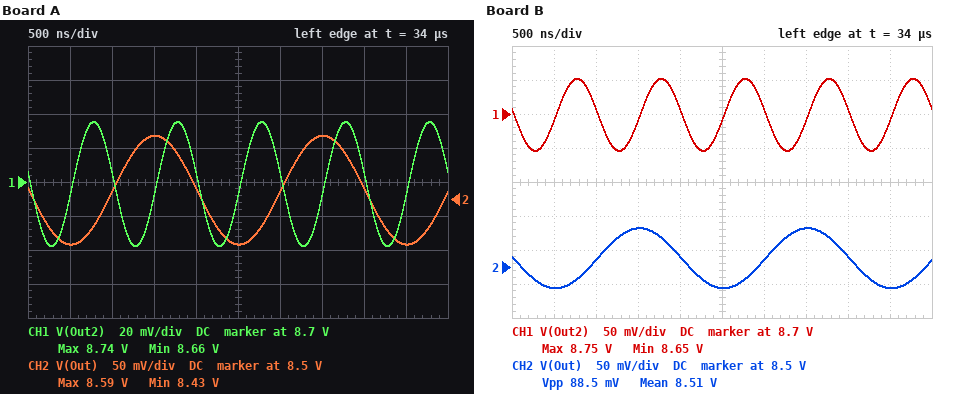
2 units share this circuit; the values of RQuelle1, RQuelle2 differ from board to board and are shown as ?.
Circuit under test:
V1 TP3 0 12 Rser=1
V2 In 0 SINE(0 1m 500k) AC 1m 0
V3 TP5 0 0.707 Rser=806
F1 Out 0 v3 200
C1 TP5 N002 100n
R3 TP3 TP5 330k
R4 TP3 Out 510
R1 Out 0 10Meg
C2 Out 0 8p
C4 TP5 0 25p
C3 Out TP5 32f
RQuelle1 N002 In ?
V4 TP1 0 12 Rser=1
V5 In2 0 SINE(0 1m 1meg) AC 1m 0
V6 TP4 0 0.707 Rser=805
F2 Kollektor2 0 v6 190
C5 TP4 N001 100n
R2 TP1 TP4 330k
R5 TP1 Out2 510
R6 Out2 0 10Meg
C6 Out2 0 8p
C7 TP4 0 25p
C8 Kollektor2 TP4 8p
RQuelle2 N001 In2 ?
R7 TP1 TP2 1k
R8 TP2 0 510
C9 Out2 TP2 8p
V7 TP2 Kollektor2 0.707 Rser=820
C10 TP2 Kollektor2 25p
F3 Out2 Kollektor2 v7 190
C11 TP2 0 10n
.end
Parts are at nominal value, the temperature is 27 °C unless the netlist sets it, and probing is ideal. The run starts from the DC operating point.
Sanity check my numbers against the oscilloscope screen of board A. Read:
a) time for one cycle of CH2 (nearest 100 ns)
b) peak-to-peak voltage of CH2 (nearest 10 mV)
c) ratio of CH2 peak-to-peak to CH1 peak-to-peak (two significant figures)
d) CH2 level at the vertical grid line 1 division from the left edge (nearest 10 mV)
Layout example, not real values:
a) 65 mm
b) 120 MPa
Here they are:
a) 2.0 µs
b) 160 mV
c) 2.2
d) 8.43 V
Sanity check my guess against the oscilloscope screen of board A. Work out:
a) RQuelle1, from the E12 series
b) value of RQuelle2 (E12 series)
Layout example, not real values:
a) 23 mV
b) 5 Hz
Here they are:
a) 470 Ω
b) 1.8 kΩ
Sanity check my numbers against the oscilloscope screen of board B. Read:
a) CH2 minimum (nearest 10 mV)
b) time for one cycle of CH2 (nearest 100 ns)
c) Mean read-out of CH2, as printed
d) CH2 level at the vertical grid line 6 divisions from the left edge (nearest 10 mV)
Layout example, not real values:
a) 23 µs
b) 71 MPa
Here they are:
a) 8.47 V
b) 2.0 µs
c) 8.51 V
d) 8.51 V
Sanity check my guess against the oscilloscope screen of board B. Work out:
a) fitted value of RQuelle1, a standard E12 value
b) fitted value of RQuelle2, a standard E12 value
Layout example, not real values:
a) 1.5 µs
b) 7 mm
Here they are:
a) 1.5 kΩ
b) 1 kΩ
